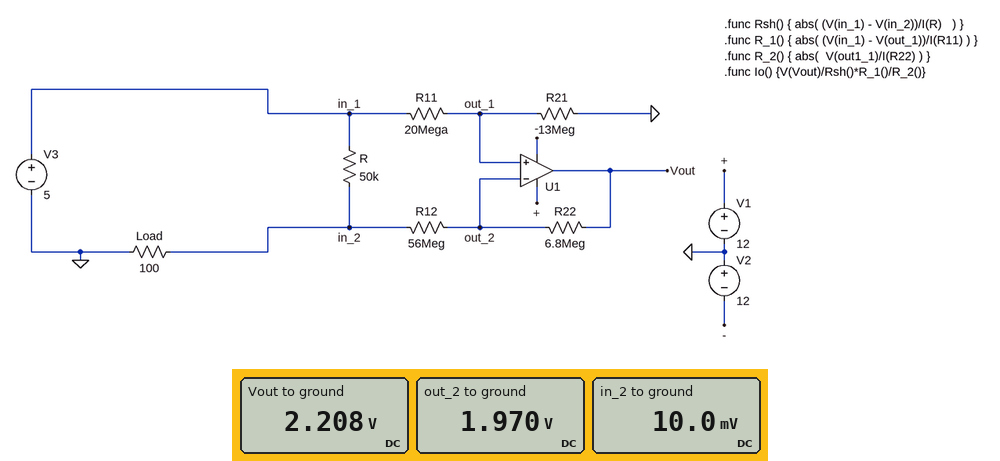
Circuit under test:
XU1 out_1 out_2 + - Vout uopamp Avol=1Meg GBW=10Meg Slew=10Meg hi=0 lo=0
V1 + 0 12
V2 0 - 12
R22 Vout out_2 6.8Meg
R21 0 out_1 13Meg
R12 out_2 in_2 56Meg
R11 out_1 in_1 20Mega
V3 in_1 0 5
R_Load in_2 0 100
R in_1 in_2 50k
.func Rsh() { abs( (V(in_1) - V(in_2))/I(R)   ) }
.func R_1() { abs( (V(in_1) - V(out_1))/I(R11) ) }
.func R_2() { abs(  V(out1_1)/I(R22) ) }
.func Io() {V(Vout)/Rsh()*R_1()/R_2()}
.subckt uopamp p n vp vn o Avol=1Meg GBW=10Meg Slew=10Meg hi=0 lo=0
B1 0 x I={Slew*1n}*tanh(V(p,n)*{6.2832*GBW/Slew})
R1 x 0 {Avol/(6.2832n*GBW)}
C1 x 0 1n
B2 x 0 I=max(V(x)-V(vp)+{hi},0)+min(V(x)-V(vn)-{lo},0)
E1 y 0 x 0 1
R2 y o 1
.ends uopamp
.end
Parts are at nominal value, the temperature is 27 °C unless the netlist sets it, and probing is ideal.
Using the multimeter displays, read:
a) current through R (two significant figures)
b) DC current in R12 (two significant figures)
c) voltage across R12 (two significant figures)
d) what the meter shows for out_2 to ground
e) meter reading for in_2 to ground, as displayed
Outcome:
100 µA
35 nA
2.0 V
1.970 V
10.0 mV
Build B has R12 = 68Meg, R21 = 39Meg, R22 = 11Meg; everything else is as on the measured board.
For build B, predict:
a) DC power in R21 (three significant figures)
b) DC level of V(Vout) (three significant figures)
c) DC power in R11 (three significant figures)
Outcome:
280 nW
3.84 V
144 nW
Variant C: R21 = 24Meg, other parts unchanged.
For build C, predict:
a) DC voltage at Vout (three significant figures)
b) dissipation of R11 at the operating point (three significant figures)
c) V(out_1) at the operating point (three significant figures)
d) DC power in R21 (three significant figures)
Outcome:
3.06 V
258 nW
2.73 V
310 nW
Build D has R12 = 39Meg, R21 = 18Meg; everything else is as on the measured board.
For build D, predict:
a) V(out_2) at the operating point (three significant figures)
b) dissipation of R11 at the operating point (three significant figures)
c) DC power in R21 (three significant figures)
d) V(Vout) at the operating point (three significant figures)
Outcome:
2.37 V
346 nW
312 nW
2.78 V
